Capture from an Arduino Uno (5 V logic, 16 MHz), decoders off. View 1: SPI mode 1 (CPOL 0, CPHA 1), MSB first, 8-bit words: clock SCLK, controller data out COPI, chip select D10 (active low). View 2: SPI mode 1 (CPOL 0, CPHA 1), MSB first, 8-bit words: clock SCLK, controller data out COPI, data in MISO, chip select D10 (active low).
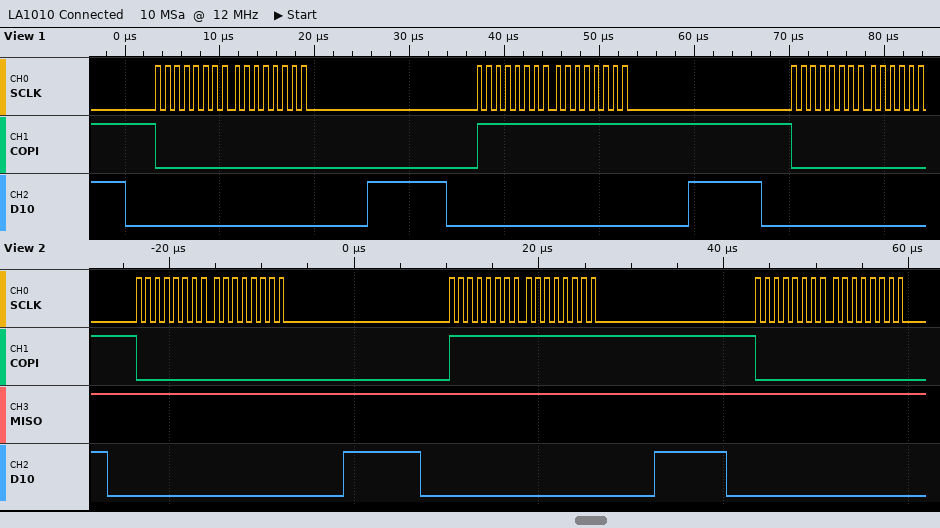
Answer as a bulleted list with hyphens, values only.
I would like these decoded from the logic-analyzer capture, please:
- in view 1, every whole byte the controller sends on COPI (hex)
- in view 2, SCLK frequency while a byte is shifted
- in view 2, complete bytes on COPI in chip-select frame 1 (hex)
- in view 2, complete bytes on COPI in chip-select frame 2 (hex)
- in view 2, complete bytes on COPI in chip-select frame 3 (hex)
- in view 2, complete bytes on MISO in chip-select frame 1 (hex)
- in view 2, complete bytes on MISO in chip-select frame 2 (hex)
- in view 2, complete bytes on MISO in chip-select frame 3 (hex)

- 0x00 0x00 0xFF 0xFF 0x00
- 1 MHz
- 0x00 0x00
- 0xFF 0xFF
- 0x00 0x00
- 0xFF 0xFF
- 0xFF 0xFF
- 0xFF 0xFF
